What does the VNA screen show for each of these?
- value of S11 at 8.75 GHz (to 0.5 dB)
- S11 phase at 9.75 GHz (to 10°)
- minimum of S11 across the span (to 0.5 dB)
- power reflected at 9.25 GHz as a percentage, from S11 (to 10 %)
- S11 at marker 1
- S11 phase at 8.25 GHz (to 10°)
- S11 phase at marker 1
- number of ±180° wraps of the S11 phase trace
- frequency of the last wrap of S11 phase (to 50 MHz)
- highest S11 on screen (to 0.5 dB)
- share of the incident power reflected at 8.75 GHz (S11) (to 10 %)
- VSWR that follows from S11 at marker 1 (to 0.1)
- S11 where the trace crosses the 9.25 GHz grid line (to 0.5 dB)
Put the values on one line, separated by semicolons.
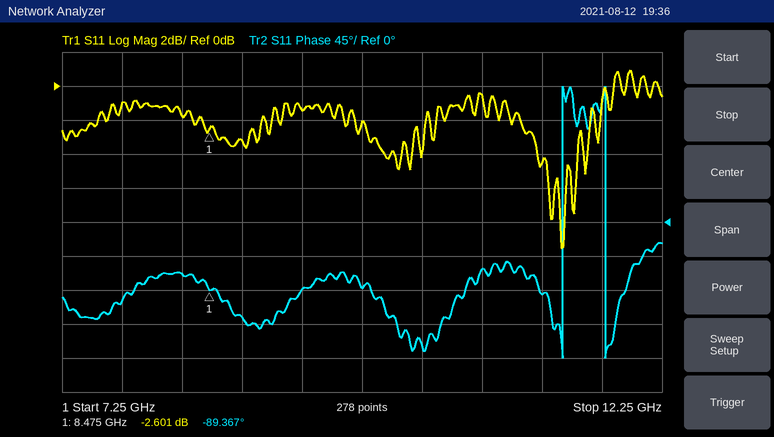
-3.0 dB; -90°; -9.5 dB; 70 %; -2.601 dB; -70°; -89.367°; 2; 11.80 GHz; 1.0 dB; 50 %; 6.7; -1.5 dB
